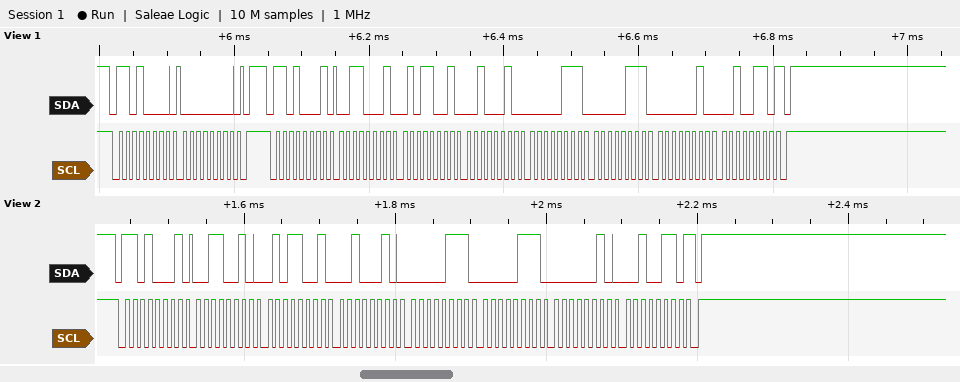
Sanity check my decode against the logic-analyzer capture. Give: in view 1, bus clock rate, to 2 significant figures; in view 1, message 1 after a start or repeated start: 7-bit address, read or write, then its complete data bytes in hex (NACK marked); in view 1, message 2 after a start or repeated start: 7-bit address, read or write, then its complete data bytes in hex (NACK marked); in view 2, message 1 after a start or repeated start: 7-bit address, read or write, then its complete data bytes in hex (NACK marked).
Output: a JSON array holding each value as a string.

["100 kHz", "0x68 write: 00", "0x68 read: 31 59 22 07 07 02 26 NACK", "0x68 read: 32 59 22 07 07 02 26 NACK"]
